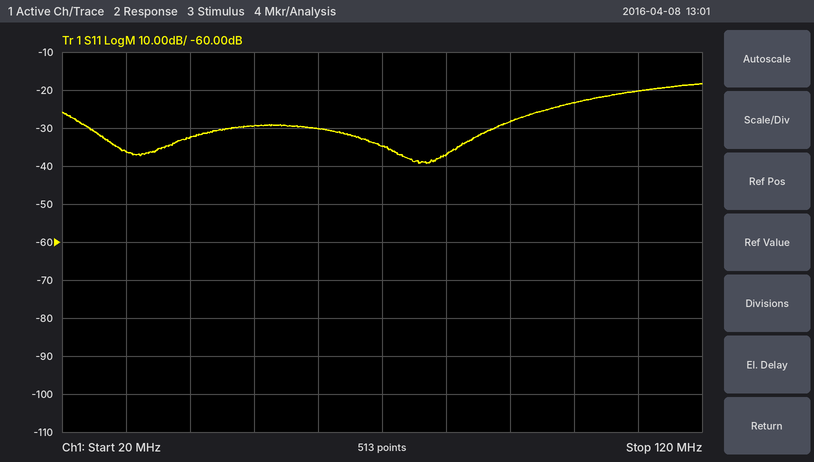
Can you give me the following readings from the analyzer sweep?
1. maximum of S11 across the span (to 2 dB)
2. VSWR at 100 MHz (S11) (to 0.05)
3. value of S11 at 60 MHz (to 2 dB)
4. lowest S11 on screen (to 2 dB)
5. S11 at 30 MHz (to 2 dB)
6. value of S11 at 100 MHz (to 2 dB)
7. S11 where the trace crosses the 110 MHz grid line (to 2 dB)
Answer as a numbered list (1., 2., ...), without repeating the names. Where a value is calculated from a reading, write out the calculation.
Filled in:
1. -18 dB
2. |Γ| = 10^(-24/20) = 0.0631; VSWR = (1 + 0.0631)/(1 − 0.0631) ≈ 1.13, so 1.15 to the nearest 0.05
3. -30 dB
4. -40 dB
5. -36 dB
6. -24 dB
7. -20 dB
